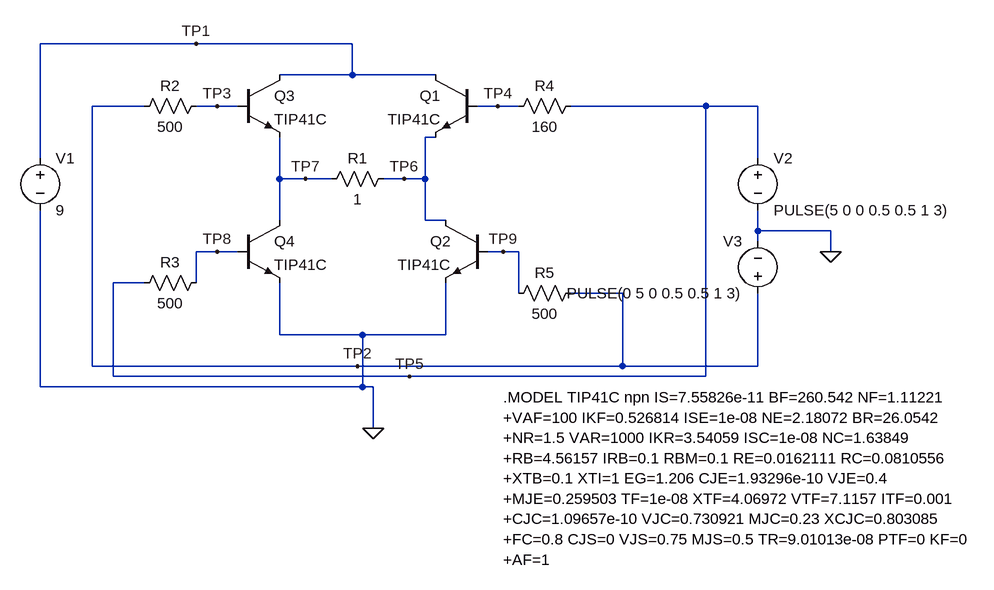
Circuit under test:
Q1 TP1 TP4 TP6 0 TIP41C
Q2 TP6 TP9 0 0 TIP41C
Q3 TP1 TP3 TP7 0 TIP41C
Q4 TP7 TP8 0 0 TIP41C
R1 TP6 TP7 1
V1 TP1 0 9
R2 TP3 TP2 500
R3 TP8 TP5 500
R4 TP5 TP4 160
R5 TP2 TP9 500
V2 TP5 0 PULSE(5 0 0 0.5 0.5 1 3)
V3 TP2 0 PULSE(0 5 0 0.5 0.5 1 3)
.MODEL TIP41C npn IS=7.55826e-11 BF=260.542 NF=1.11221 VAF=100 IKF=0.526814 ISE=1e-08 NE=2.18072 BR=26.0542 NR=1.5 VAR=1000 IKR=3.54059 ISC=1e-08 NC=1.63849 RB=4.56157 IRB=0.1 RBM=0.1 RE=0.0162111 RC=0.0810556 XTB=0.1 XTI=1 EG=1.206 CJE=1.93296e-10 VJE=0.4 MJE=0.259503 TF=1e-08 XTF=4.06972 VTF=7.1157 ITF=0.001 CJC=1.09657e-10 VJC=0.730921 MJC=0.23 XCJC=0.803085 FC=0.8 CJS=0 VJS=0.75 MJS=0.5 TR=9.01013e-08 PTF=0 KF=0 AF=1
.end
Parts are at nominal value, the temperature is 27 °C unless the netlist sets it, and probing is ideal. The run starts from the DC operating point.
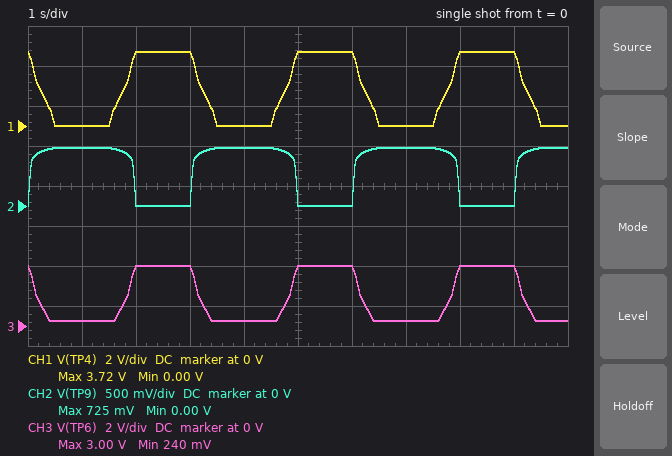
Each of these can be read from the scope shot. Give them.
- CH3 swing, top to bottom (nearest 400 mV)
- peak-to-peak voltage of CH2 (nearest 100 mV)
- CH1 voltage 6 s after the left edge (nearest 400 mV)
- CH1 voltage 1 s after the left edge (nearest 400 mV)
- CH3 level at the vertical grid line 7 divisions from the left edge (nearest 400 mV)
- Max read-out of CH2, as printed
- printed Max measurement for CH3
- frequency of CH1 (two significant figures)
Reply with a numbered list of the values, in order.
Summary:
1. 2.8 V
2. 700 mV
3. 3.6 V
4. 0 V
5. 400 mV
6. 725 mV
7. 3.00 V
8. 330 mHz
